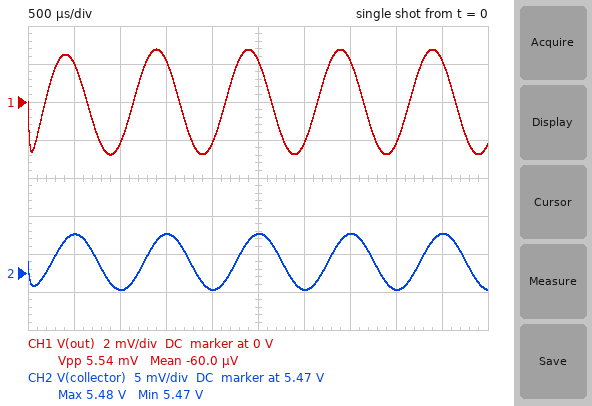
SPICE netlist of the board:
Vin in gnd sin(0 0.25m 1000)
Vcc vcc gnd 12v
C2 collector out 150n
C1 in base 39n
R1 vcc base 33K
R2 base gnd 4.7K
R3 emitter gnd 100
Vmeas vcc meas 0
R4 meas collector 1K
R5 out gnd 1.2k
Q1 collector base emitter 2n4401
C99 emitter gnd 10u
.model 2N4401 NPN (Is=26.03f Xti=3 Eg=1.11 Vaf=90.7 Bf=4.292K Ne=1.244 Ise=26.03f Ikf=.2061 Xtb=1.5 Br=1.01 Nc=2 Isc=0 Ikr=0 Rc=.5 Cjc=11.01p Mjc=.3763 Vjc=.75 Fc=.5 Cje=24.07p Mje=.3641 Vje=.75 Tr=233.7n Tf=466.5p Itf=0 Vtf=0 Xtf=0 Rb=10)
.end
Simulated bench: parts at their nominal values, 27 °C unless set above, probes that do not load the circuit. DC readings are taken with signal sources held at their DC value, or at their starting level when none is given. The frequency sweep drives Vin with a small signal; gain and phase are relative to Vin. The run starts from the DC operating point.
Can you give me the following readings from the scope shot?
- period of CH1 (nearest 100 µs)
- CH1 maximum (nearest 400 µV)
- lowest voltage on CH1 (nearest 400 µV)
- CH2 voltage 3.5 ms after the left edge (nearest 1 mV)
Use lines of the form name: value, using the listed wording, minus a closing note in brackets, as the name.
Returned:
period of CH1: 1.0 ms
CH1 maximum: 2.8 mV
lowest voltage on CH1: -2.8 mV
CH2 voltage 3.5 ms after the left edge: 5.475 V
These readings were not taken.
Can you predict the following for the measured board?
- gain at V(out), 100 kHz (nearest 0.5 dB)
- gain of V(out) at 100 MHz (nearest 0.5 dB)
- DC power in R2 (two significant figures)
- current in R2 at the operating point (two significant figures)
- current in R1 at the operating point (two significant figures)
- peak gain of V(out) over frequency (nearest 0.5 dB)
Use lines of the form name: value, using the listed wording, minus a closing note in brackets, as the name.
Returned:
gain at V(out), 100 kHz: 42.0 dB
gain of V(out) at 100 MHz: 25.0 dB
DC power in R2: 380 µW
current in R2 at the operating point: 280 µA
current in R1 at the operating point: 320 µA
peak gain of V(out) over frequency: 42.0 dB
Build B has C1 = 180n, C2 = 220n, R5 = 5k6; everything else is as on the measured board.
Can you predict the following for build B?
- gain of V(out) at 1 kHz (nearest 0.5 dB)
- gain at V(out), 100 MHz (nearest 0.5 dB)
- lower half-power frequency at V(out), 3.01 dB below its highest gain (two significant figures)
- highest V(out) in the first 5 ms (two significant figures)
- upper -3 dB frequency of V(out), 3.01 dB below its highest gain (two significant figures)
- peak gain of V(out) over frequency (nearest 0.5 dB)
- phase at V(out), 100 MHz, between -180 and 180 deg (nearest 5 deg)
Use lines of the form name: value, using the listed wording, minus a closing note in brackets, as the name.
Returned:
gain of V(out) at 1 kHz: 31.5 dB
gain at V(out), 100 MHz: 25.5 dB
lower half-power frequency at V(out), 3.01 dB below its highest gain: 4.9 kHz
highest V(out) in the first 5 ms: 9.6 mV
upper -3 dB frequency of V(out), 3.01 dB below its highest gain: 10 MHz
peak gain of V(out) over frequency: 45.5 dB
phase at V(out), 100 MHz, between -180 and 180 deg: 80 deg
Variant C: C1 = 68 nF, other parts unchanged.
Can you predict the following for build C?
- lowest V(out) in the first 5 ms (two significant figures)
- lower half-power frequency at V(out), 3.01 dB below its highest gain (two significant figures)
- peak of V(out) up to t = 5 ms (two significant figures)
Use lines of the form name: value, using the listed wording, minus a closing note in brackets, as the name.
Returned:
lowest V(out) in the first 5 ms: -3.9 mV
lower half-power frequency at V(out), 3.01 dB below its highest gain: 6.9 kHz
peak of V(out) up to t = 5 ms: 3.9 mV
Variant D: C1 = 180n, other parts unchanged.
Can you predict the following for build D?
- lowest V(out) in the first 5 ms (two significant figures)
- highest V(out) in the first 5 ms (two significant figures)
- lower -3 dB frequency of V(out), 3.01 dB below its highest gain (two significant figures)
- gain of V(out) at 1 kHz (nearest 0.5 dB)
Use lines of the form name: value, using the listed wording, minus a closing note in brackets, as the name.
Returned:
lowest V(out) in the first 5 ms: -5.7 mV
highest V(out) in the first 5 ms: 5.6 mV
lower -3 dB frequency of V(out), 3.01 dB below its highest gain: 5.0 kHz
gain of V(out) at 1 kHz: 27.0 dB
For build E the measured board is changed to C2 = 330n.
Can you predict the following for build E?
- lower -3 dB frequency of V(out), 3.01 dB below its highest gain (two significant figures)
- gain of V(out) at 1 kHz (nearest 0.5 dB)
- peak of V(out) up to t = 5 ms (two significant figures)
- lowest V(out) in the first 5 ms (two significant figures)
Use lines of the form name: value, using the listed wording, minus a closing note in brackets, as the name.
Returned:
lower -3 dB frequency of V(out), 3.01 dB below its highest gain: 9.1 kHz
gain of V(out) at 1 kHz: 21.5 dB
peak of V(out) up to t = 5 ms: 3.0 mV
lowest V(out) in the first 5 ms: -3.0 mV
